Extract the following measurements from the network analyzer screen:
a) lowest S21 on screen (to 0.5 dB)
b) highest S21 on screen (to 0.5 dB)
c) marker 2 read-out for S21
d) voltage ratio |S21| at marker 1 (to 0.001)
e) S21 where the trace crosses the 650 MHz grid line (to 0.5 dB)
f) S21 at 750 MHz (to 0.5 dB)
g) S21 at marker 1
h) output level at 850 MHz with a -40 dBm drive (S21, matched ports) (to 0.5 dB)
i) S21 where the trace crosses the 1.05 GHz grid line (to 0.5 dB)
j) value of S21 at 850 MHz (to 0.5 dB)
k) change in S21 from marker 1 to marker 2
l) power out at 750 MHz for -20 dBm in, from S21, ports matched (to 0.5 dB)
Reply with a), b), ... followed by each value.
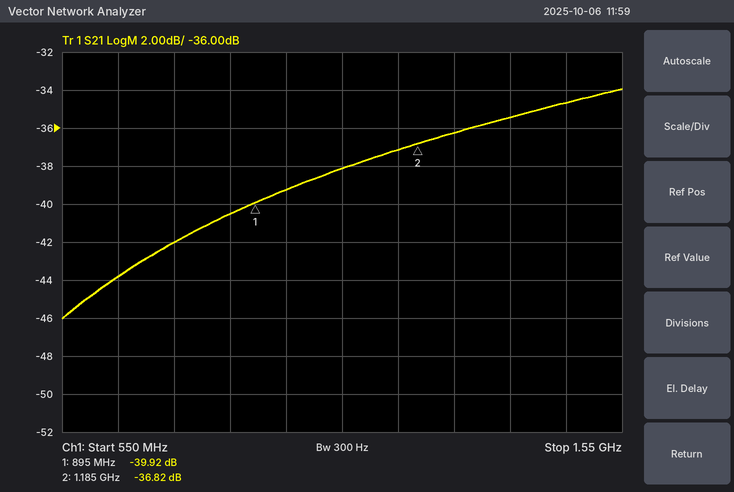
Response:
a) -46.0 dB
b) -34.0 dB
c) -36.82 dB
d) 0.010
e) -44.0 dB
f) -42.0 dB
g) -39.92 dB
h) -80.5 dBm
i) -38.0 dB
j) -40.5 dB
k) 3.10 dB
l) -62.0 dBm
